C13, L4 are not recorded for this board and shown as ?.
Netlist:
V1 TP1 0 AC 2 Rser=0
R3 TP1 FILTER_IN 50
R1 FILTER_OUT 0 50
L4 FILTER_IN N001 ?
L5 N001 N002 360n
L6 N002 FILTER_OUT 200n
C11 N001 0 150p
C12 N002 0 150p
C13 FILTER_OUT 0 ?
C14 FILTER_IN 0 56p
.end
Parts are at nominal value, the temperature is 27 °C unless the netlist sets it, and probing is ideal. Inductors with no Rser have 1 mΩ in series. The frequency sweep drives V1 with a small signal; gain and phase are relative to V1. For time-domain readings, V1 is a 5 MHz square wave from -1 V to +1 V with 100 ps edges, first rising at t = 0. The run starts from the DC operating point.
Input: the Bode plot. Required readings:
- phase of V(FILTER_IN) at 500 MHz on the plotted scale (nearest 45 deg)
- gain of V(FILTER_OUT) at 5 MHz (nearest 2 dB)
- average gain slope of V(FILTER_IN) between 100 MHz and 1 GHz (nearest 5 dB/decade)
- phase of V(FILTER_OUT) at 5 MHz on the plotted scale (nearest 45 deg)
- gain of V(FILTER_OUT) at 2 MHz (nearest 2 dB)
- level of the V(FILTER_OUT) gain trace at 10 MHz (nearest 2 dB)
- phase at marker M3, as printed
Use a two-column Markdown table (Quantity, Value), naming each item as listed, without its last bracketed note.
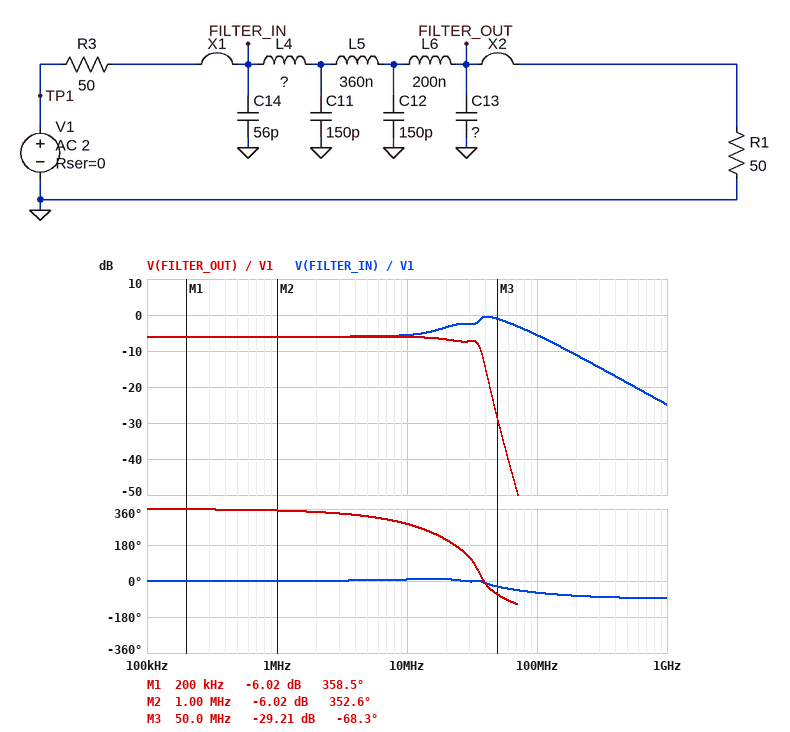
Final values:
| Quantity | Value |
|---|---|
| phase of V(FILTER_IN) at 500 MHz on the plotted scale | -90 deg |
| gain of V(FILTER_OUT) at 5 MHz | -6 dB |
| average gain slope of V(FILTER_IN) between 100 MHz and 1 GHz | -20 dB/decade |
| phase of V(FILTER_OUT) at 5 MHz on the plotted scale | 315 deg |
| gain of V(FILTER_OUT) at 2 MHz | -6 dB |
| level of the V(FILTER_OUT) gain trace at 10 MHz | -6 dB |
| phase at marker M3, as printed | -68.3 deg |
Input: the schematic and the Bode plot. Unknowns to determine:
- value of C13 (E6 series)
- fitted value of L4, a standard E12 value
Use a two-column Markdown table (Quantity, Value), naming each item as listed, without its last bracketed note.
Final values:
| Quantity | Value |
|---|---|
| value of C13 | 15 pF |
| fitted value of L4, a standard E12 value | 560 nH |
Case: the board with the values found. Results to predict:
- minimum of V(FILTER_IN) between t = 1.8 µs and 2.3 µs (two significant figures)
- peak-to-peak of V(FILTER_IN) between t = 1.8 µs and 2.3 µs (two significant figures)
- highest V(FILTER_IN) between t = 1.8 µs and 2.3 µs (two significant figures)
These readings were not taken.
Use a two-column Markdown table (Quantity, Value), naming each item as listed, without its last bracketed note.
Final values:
| Quantity | Value |
|---|---|
| minimum of V(FILTER_IN) between t = 1.8 µs and 2.3 µs | -980 mV |
| peak-to-peak of V(FILTER_IN) between t = 1.8 µs and 2.3 µs | 2.0 V |
| highest V(FILTER_IN) between t = 1.8 µs and 2.3 µs | 980 mV |
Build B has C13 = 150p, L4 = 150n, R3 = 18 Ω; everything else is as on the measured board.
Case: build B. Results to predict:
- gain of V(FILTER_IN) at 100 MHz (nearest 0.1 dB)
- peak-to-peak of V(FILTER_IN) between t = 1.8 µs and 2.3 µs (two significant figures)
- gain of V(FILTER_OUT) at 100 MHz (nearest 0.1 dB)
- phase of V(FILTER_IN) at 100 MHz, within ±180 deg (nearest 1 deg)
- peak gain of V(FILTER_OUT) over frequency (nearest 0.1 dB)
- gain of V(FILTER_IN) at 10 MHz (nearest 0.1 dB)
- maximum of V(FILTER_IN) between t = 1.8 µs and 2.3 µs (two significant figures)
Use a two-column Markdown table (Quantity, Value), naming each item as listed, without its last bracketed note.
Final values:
| Quantity | Value |
|---|---|
| gain of V(FILTER_IN) at 100 MHz | -0.7 dB |
| peak-to-peak of V(FILTER_IN) between t = 1.8 µs and 2.3 µs | 1.8 V |
| gain of V(FILTER_OUT) at 100 MHz | -64.3 dB |
| phase of V(FILTER_IN) at 100 MHz, within ±180 deg | -23 deg |
| peak gain of V(FILTER_OUT) over frequency | -1.6 dB |
| gain of V(FILTER_IN) at 10 MHz | -3.8 dB |
| maximum of V(FILTER_IN) between t = 1.8 µs and 2.3 µs | 890 mV |
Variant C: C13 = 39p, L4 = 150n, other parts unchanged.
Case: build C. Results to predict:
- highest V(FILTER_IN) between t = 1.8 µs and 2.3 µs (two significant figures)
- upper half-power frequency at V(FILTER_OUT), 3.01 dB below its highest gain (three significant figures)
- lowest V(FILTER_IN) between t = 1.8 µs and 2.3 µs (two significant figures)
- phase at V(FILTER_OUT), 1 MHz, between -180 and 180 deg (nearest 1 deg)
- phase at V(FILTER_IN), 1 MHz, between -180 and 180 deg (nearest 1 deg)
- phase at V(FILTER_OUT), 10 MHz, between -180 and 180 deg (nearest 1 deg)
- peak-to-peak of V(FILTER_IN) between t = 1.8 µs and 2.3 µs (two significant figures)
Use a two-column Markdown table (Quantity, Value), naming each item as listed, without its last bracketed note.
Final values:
| Quantity | Value |
|---|---|
| highest V(FILTER_IN) between t = 1.8 µs and 2.3 µs | 720 mV |
| upper half-power frequency at V(FILTER_OUT), 3.01 dB below its highest gain | 37.9 MHz |
| lowest V(FILTER_IN) between t = 1.8 µs and 2.3 µs | -720 mV |
| phase at V(FILTER_OUT), 1 MHz, between -180 and 180 deg | -6 deg |
| phase at V(FILTER_IN), 1 MHz, between -180 and 180 deg | -1 deg |
| phase at V(FILTER_OUT), 10 MHz, between -180 and 180 deg | -61 deg |
| peak-to-peak of V(FILTER_IN) between t = 1.8 µs and 2.3 µs | 1.4 V |
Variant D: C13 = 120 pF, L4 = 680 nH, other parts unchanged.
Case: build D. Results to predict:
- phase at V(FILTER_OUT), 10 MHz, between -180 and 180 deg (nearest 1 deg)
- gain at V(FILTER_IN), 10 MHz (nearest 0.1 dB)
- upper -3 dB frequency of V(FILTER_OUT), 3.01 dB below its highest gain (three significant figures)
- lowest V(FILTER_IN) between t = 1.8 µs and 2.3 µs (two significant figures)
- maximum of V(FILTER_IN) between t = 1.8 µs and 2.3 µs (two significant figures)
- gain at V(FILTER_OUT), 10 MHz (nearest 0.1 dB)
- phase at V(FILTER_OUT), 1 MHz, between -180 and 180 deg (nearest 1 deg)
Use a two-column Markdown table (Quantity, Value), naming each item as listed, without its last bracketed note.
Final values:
| Quantity | Value |
|---|---|
| phase at V(FILTER_OUT), 10 MHz, between -180 and 180 deg | -90 deg |
| gain at V(FILTER_IN), 10 MHz | -5.0 dB |
| upper -3 dB frequency of V(FILTER_OUT), 3.01 dB below its highest gain | 30.7 MHz |
| lowest V(FILTER_IN) between t = 1.8 µs and 2.3 µs | -1.0 V |
| maximum of V(FILTER_IN) between t = 1.8 µs and 2.3 µs | 1.0 V |
| gain at V(FILTER_OUT), 10 MHz | -6.6 dB |
| phase at V(FILTER_OUT), 1 MHz, between -180 and 180 deg | -9 deg |
